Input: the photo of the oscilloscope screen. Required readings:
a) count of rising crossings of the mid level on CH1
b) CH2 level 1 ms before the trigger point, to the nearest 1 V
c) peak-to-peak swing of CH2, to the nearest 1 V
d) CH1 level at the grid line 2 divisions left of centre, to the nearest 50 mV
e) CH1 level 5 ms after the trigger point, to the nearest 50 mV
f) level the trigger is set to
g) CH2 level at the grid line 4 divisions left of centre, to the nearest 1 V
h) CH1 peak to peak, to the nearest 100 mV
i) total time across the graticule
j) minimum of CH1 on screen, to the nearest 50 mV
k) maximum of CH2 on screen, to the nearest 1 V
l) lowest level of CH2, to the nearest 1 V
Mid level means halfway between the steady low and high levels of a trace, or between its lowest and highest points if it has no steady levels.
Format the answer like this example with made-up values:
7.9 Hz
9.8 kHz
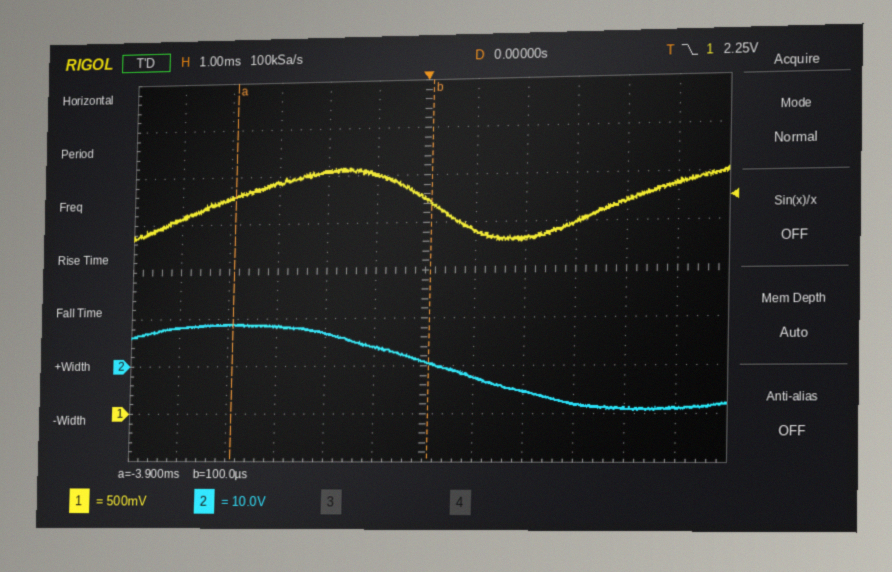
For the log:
2
4 V
18 V
2.55 V
2.40 V
2.25 V
9 V
800 mV
12 ms
1.80 V
9 V
-9 V
